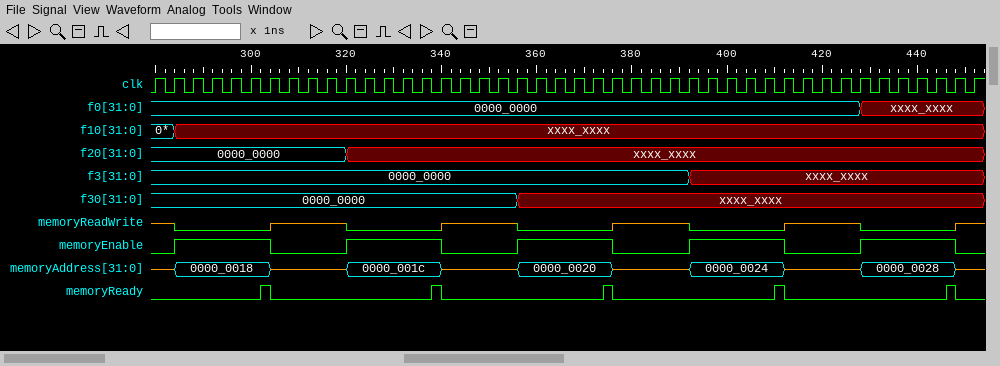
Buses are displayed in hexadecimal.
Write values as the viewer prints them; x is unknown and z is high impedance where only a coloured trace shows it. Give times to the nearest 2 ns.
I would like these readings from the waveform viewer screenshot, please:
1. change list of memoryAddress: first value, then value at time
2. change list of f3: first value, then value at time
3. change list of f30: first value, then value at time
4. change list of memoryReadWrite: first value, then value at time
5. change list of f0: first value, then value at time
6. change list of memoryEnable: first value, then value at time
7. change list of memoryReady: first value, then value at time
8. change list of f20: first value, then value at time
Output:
z, 0000_0018 at 284 ns, z at 304 ns, 0000_001c at 320 ns, z at 340 ns, 0000_0020 at 356 ns, z at 376 ns, 0000_0024 at 392 ns, z at 412 ns, 0000_0028 at 428 ns, z at 448 ns
0000_0000, xxxx_xxxx at 392 ns
0000_0000, xxxx_xxxx at 356 ns
z, 0 at 284 ns, z at 304 ns, 0 at 320 ns, z at 340 ns, 0 at 356 ns, z at 376 ns, 0 at 392 ns, z at 412 ns, 0 at 428 ns, z at 448 ns
0000_0000, xxxx_xxxx at 428 ns
0, 1 at 284 ns, 0 at 304 ns, 1 at 320 ns, 0 at 340 ns, 1 at 356 ns, 0 at 376 ns, 1 at 392 ns, 0 at 412 ns, 1 at 428 ns, 0 at 448 ns
0, 1 at 302 ns, 0 at 304 ns, 1 at 338 ns, 0 at 340 ns, 1 at 374 ns, 0 at 376 ns, 1 at 410 ns, 0 at 412 ns, 1 at 446 ns, 0 at 448 ns
0000_0000, xxxx_xxxx at 320 ns
